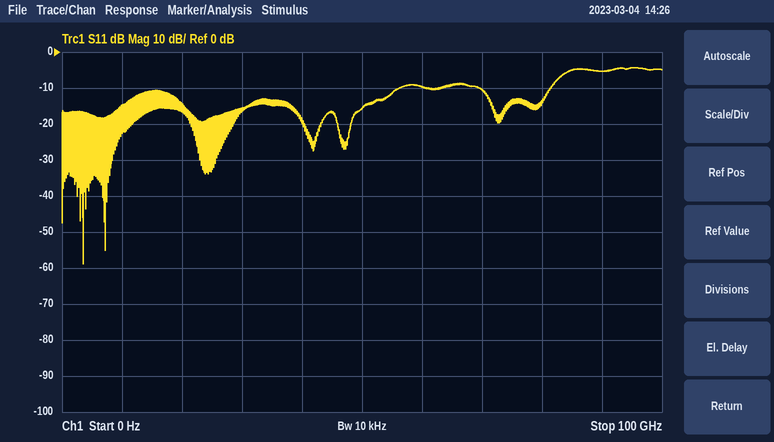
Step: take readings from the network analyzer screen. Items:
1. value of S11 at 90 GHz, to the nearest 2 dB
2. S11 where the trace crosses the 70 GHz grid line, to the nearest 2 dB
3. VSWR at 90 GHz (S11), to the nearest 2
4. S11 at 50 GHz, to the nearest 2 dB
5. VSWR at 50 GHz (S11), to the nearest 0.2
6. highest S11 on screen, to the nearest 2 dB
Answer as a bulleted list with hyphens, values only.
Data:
- -6 dB
- -10 dB
- 4
- -16 dB
- 1.4
- -4 dB
